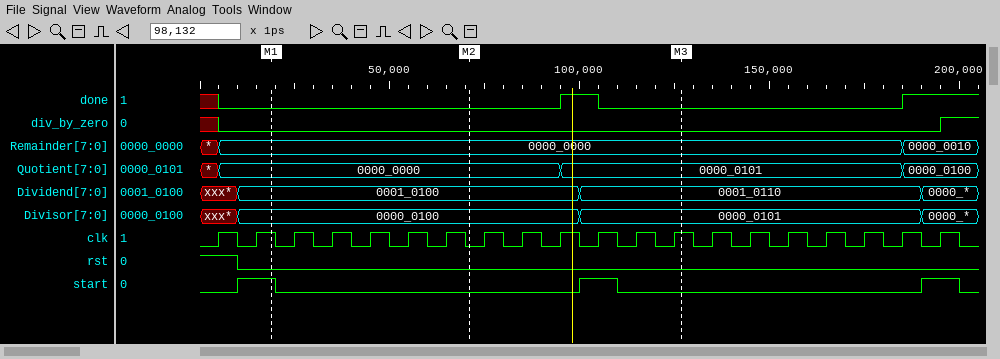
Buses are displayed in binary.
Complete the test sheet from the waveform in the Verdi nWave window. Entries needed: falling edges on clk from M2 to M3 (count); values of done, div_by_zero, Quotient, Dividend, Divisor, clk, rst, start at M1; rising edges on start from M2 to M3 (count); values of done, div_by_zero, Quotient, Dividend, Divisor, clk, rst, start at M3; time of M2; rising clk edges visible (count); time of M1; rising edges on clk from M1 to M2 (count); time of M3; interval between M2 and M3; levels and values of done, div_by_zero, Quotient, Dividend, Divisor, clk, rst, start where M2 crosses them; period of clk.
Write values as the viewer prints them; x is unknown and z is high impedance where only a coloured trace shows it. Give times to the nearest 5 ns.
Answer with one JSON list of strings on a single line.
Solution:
["5", "done=0, div_by_zero=0, Quotient=0000_0000, Dividend=0001_0100, Divisor=0000_0100, clk=1, rst=0, start=1", "1", "done=0, div_by_zero=0, Quotient=0000_0101, Dividend=0001_0110, Divisor=0000_0101, clk=1, rst=0, start=0", "70 ns", "20", "20 ns", "5", "125 ns", "55 ns", "done=0, div_by_zero=0, Quotient=0000_0000, Dividend=0001_0100, Divisor=0000_0100, clk=0, rst=0, start=0", "10 ns"]
